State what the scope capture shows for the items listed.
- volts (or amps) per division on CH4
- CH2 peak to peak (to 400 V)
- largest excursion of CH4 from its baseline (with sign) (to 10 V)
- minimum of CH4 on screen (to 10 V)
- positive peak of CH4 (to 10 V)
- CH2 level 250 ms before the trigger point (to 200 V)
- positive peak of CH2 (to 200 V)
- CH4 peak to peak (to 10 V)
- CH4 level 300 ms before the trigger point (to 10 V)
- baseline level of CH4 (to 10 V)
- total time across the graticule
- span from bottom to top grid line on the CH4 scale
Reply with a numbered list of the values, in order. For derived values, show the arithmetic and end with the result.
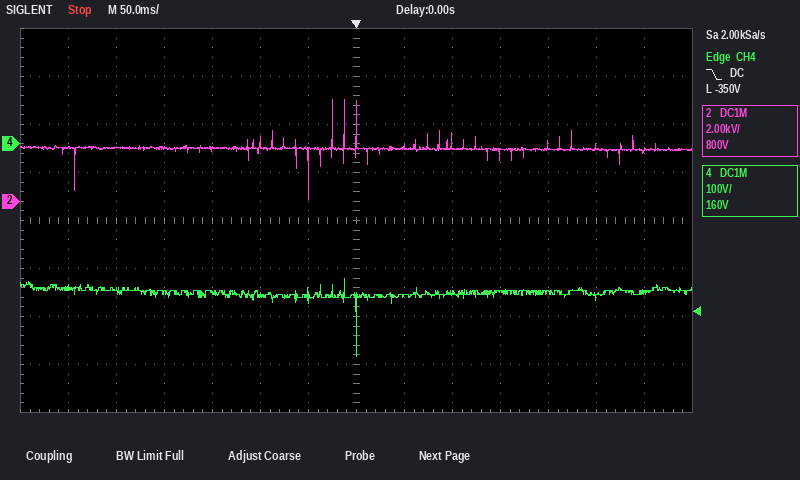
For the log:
1. 100 V
2. 4.0 kV
3. -440 V − (-310 V) = -130 V
4. -440 V
5. -280 V
6. 2.2 kV
7. 4.2 kV
8. -280 V − (-440 V) = 160 V
9. -300 V
10. -310 V
11. 700 ms
12. 800 V
